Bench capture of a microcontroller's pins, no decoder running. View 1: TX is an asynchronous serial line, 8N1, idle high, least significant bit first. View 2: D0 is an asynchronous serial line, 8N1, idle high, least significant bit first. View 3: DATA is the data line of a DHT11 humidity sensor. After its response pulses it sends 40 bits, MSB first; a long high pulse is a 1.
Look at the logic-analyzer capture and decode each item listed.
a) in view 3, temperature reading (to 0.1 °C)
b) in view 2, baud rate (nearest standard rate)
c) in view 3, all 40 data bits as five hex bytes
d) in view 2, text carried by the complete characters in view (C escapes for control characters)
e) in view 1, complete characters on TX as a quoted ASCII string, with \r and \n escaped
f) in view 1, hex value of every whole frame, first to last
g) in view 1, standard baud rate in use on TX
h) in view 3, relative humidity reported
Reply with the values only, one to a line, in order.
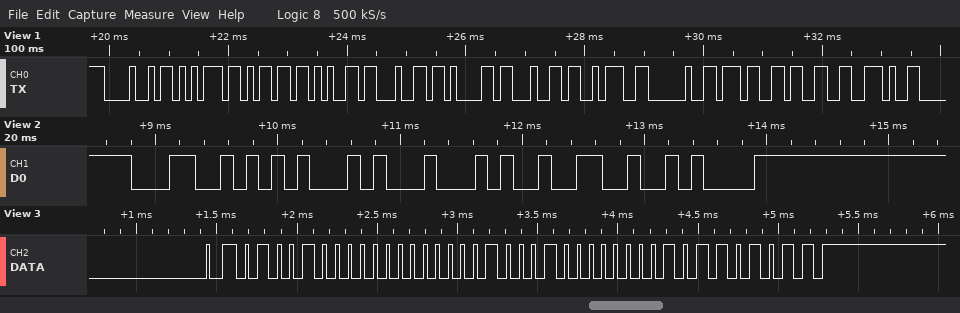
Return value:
34.1 °C
9600 baud
48 00 22 01 6B
"LED2\n"
"Humedad: 73."
0x48 0x75 0x6D 0x65 0x64 0x61 0x64 0x3A 0x20 0x37 0x33 0x2E
9600 baud
72 %
